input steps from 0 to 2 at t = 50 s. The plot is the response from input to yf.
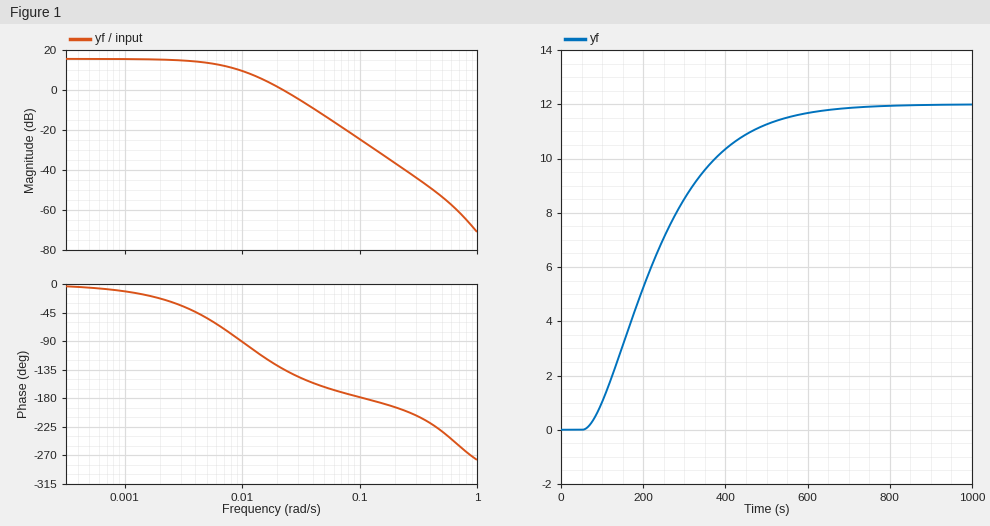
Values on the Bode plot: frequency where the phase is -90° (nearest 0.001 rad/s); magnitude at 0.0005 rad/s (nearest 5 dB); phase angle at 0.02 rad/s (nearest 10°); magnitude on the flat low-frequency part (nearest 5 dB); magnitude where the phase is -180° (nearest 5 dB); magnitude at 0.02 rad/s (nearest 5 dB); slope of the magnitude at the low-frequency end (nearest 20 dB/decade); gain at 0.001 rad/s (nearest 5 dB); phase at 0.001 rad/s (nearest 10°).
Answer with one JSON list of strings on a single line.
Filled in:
["0.010 rad/s", "15 dB", "-130°", "15 dB", "-25 dB", "0 dB", "0 dB/decade", "15 dB", "-10°"]
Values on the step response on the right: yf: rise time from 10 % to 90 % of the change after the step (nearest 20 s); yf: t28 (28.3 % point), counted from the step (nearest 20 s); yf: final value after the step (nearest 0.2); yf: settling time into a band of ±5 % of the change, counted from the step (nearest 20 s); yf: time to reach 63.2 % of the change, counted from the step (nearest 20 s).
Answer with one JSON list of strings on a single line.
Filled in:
["340 s", "100 s", "12.0", "480 s", "220 s"]
